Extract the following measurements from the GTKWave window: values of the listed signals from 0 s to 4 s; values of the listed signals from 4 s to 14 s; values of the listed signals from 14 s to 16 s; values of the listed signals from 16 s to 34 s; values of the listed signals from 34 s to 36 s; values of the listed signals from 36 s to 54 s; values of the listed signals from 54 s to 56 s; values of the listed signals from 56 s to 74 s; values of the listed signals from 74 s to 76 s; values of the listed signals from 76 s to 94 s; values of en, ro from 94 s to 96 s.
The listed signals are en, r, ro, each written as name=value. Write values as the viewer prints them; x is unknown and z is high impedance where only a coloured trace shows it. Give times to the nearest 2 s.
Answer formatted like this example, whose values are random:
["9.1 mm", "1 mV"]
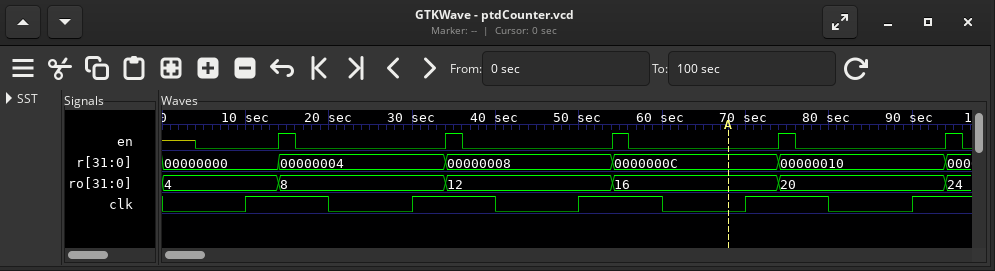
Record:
["en=z, r=00000000, ro=4", "en=0, r=00000000, ro=4", "en=1, r=00000004, ro=8", "en=0, r=00000004, ro=8", "en=1, r=00000008, ro=12", "en=0, r=00000008, ro=12", "en=1, r=0000000C, ro=16", "en=0, r=0000000C, ro=16", "en=1, r=00000010, ro=20", "en=0, r=00000010, ro=20", "en=1, ro=24"]
